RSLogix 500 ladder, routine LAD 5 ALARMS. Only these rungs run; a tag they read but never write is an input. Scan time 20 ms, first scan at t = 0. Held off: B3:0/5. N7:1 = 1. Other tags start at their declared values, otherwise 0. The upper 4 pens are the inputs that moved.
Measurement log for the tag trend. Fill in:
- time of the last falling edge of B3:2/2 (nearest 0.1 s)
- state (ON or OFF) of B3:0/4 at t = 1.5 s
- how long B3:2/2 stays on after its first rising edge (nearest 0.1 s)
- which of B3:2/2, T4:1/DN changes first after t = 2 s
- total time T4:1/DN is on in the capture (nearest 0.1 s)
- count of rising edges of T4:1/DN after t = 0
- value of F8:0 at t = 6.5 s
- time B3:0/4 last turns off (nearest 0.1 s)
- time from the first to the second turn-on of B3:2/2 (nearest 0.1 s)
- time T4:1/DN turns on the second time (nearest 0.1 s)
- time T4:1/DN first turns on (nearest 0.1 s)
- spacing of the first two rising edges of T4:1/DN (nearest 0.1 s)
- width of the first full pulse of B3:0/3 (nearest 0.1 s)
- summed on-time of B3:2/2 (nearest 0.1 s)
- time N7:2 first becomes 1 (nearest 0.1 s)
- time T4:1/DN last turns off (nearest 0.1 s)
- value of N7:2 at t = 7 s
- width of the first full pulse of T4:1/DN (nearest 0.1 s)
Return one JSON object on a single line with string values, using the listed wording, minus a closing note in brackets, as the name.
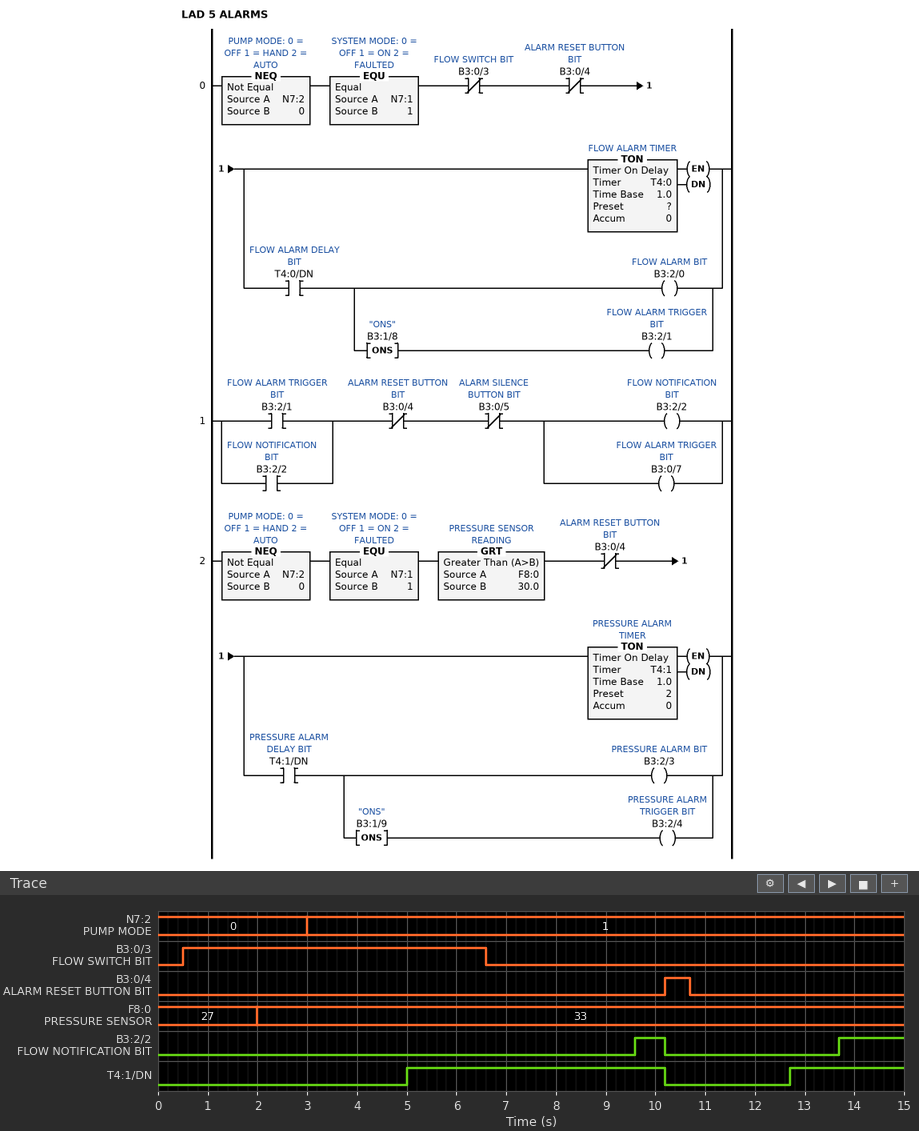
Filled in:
{"time of the last falling edge of B3:2/2": "10.2 s", "state (ON or OFF) of B3:0/4 at t = 1.5 s": "OFF", "how long B3:2/2 stays on after its first rising edge": "0.6 s", "which of B3:2/2, T4:1/DN changes first after t = 2 s": "T4:1/DN", "total time T4:1/DN is on in the capture": "7.5 s", "count of rising edges of T4:1/DN after t = 0": "2", "value of F8:0 at t = 6.5 s": "33", "time B3:0/4 last turns off": "10.7 s", "time from the first to the second turn-on of B3:2/2": "4.1 s", "time T4:1/DN turns on the second time": "12.7 s", "time T4:1/DN first turns on": "5.0 s", "spacing of the first two rising edges of T4:1/DN": "7.7 s", "width of the first full pulse of B3:0/3": "6.1 s", "summed on-time of B3:2/2": "1.9 s", "time N7:2 first becomes 1": "3.0 s", "time T4:1/DN last turns off": "10.2 s", "value of N7:2 at t = 7 s": "1", "width of the first full pulse of T4:1/DN": "5.2 s"}
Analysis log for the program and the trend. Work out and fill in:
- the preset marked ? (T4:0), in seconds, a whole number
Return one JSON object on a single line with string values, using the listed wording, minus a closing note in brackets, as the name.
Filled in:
{"the preset marked ? (T4:0), in seconds, a whole number": "3 s"}
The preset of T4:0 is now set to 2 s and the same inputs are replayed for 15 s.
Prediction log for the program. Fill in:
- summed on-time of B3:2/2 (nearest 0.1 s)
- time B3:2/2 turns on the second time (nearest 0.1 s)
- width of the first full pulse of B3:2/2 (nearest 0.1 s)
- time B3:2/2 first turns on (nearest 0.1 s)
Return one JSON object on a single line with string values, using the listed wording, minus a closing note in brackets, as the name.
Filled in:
{"summed on-time of B3:2/2": "3.9 s", "time B3:2/2 turns on the second time": "12.7 s", "width of the first full pulse of B3:2/2": "1.6 s", "time B3:2/2 first turns on": "8.6 s"}
